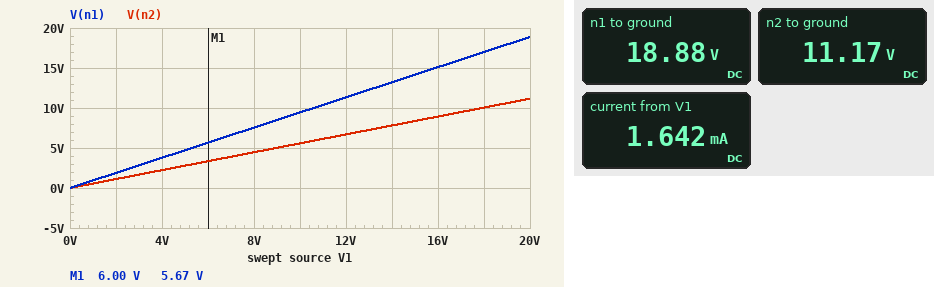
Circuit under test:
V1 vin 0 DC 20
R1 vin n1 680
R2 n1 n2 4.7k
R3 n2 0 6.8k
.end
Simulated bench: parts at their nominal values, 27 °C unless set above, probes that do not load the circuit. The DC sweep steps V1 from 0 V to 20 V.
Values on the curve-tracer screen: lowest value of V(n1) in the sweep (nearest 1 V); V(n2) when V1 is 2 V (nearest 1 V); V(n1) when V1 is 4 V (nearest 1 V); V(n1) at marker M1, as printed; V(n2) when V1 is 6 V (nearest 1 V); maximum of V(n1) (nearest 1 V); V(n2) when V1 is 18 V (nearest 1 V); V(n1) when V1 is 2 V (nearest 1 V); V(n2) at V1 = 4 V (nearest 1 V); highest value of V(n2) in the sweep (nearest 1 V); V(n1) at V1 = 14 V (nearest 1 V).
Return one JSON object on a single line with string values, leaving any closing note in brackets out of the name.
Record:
{"lowest value of V(n1) in the sweep": "0 V", "V(n2) when V1 is 2 V": "1 V", "V(n1) when V1 is 4 V": "4 V", "V(n1) at marker M1, as printed": "5.67 V", "V(n2) when V1 is 6 V": "3 V", "maximum of V(n1)": "19 V", "V(n2) when V1 is 18 V": "10 V", "V(n1) when V1 is 2 V": "2 V", "V(n2) at V1 = 4 V": "2 V", "highest value of V(n2) in the sweep": "11 V", "V(n1) at V1 = 14 V": "13 V"}
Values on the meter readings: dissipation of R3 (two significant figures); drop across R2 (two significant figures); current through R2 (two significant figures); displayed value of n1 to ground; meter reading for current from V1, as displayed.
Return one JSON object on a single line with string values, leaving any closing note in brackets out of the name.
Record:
{"dissipation of R3": "18 mW", "drop across R2": "7.7 V", "current through R2": "1.6 mA", "displayed value of n1 to ground": "18.88 V", "meter reading for current from V1, as displayed": "1.642 mA"}
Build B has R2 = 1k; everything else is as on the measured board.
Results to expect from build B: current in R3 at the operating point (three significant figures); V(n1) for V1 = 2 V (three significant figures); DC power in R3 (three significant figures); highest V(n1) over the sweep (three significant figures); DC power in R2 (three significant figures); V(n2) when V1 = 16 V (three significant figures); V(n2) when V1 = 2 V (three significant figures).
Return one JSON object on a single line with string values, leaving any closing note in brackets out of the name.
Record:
{"current in R3 at the operating point": "2.36 mA", "V(n1) for V1 = 2 V": "1.84 V", "DC power in R3": "37.8 mW", "highest V(n1) over the sweep": "18.4 V", "DC power in R2": "5.56 mW", "V(n2) when V1 = 16 V": "12.8 V", "V(n2) when V1 = 2 V": "1.60 V"}
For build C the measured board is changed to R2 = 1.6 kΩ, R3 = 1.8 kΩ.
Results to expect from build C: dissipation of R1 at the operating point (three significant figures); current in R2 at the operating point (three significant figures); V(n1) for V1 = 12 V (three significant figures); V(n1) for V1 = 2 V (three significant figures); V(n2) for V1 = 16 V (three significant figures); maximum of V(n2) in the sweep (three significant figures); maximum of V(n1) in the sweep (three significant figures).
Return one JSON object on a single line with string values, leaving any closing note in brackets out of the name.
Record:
{"dissipation of R1 at the operating point": "16.3 mW", "current in R2 at the operating point": "4.90 mA", "V(n1) for V1 = 12 V": "10.0 V", "V(n1) for V1 = 2 V": "1.67 V", "V(n2) for V1 = 16 V": "7.06 V", "maximum of V(n2) in the sweep": "8.82 V", "maximum of V(n1) in the sweep": "16.7 V"}
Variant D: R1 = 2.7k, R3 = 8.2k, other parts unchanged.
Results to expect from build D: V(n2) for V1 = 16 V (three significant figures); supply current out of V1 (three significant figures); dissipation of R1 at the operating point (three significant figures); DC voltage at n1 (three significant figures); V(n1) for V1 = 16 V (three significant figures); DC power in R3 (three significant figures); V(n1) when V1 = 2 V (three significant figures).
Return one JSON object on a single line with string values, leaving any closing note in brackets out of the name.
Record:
{"V(n2) for V1 = 16 V": "8.41 V", "supply current out of V1": "1.28 mA", "dissipation of R1 at the operating point": "4.44 mW", "DC voltage at n1": "16.5 V", "V(n1) for V1 = 16 V": "13.2 V", "DC power in R3": "13.5 mW", "V(n1) when V1 = 2 V": "1.65 V"}
